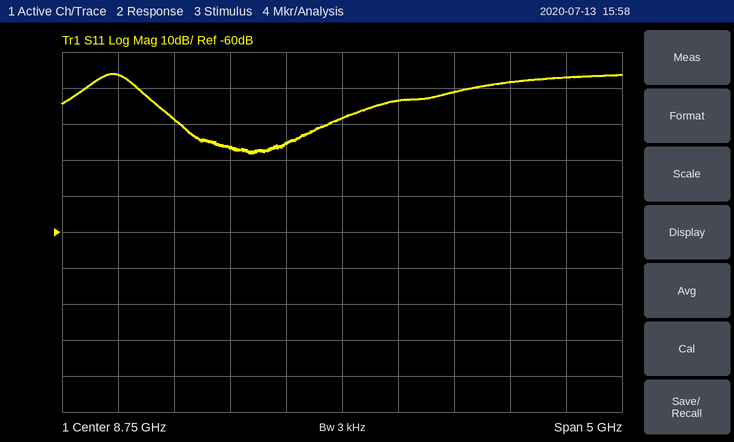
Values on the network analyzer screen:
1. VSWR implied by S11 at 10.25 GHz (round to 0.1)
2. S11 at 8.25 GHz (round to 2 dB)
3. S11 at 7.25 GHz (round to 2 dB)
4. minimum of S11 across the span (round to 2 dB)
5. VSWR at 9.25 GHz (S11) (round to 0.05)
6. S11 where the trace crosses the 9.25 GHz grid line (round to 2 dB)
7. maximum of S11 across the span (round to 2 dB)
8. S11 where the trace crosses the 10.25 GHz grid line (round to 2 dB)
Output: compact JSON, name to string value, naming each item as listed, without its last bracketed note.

{"VSWR implied by S11 at 10.25 GHz": "1.3", "S11 at 8.25 GHz": "-36 dB", "S11 at 7.25 GHz": "-28 dB", "minimum of S11 across the span": "-38 dB", "VSWR at 9.25 GHz (S11)": "1.15", "S11 where the trace crosses the 9.25 GHz grid line": "-24 dB", "maximum of S11 across the span": "-16 dB", "S11 where the trace crosses the 10.25 GHz grid line": "-18 dB"}
